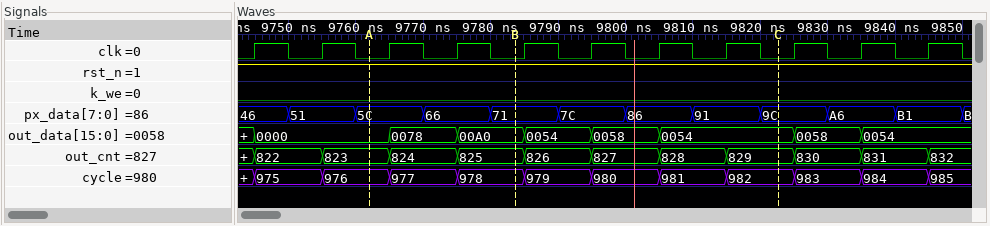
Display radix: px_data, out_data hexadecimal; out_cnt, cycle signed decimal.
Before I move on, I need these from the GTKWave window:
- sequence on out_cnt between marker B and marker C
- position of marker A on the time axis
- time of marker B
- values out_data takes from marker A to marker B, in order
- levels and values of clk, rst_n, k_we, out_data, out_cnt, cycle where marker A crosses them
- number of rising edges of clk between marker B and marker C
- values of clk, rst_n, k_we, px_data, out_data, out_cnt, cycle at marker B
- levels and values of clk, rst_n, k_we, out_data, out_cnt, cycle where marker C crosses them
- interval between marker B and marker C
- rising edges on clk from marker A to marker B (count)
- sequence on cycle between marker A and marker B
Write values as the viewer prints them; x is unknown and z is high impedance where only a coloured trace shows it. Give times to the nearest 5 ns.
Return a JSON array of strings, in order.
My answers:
["825, 826, 827, 828, 829", "9760 ns", "9785 ns", "0000, 0078, 00A0", "clk=0, rst_n=1, k_we=0, out_data=0000, out_cnt=823, cycle=976", "4", "clk=0, rst_n=1, k_we=0, px_data=71, out_data=00A0, out_cnt=825, cycle=978", "clk=0, rst_n=1, k_we=0, out_data=0054, out_cnt=829, cycle=982", "40 ns", "2", "976, 977, 978"]
